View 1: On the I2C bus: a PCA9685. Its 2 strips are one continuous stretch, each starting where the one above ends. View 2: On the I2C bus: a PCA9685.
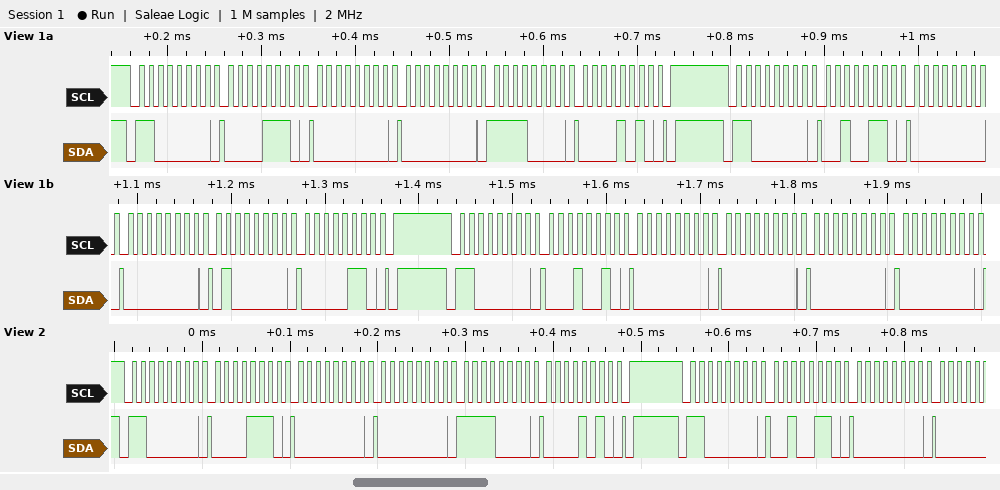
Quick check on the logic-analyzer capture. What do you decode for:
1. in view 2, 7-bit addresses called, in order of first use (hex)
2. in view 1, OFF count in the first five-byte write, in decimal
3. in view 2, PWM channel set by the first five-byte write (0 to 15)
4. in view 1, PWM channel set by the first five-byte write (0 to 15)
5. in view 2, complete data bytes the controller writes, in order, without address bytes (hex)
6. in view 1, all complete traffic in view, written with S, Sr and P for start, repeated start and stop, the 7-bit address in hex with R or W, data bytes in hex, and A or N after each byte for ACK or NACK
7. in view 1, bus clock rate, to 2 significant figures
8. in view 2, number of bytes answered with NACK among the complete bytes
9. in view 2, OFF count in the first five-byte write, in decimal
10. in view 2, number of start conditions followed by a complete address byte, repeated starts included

0x60
2800
2
2
0E 00 00 F0 0A 26 00
S 60W A 0E A 00 A 00 A F0 A 0A A P S 60W A 26 A 00 A 00 A 40 A 06 A P S 60W A 12 A 00 A 00 A 00 A 00 A
100 kHz
0
2800
2
